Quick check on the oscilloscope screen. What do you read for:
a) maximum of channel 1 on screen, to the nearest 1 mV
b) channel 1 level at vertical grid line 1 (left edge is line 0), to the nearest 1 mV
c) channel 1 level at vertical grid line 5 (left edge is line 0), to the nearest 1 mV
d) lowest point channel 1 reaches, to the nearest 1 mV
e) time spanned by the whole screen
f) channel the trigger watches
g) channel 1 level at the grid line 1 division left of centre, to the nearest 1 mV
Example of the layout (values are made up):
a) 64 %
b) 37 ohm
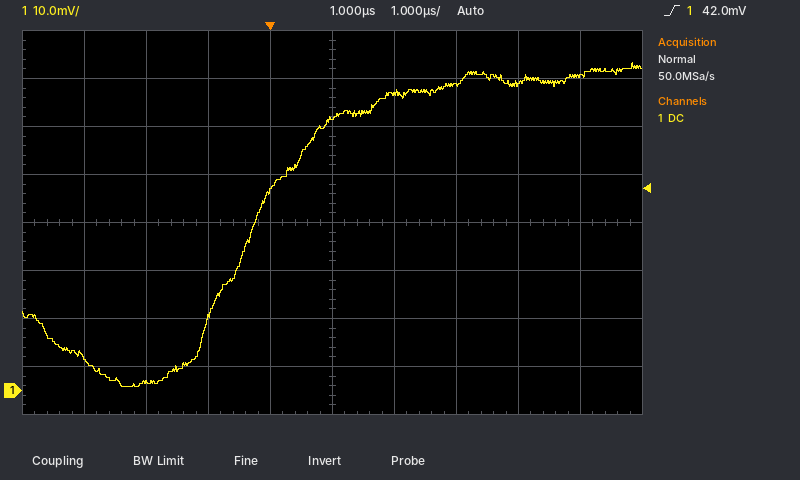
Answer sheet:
a) 68 mV
b) 7 mV
c) 57 mV
d) 1 mV
e) 10 µs
f) channel 1
g) 42 mV
